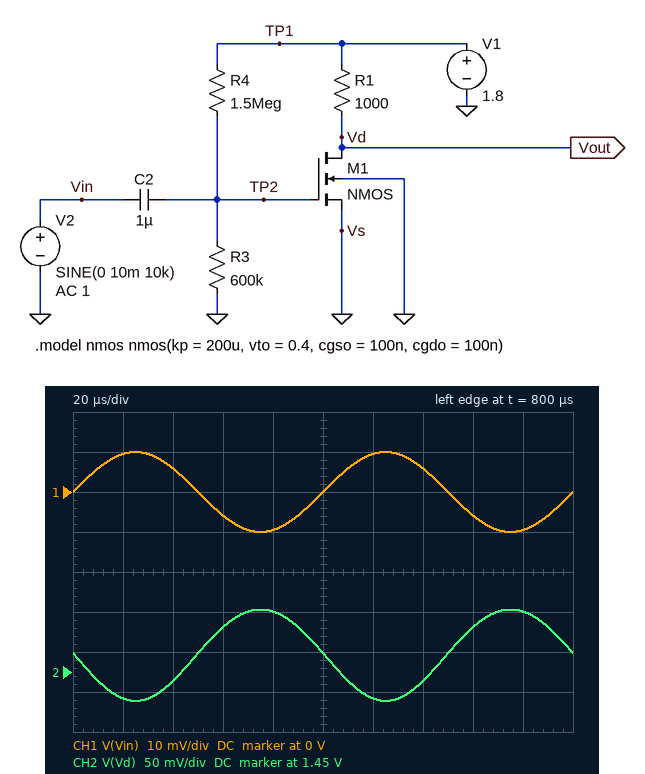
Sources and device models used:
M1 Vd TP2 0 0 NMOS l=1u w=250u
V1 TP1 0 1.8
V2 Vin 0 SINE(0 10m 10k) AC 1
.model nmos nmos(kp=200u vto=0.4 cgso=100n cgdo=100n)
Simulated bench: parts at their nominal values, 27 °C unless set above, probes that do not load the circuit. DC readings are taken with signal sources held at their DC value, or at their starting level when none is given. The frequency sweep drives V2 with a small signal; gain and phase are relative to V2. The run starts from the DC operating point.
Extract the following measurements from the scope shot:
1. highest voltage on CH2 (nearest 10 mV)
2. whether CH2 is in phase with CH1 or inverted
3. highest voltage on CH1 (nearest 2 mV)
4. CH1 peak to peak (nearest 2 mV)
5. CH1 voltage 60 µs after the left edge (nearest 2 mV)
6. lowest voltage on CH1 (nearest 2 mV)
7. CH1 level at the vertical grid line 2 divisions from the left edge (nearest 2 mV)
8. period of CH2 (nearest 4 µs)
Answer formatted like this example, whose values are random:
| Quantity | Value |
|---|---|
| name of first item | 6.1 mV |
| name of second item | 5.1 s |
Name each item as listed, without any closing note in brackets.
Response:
| Quantity | Value |
|---|---|
| highest voltage on CH2 | 1.53 V |
| whether CH2 is in phase with CH1 or inverted | inverted |
| highest voltage on CH1 | 10 mV |
| CH1 peak to peak | 20 mV |
| CH1 voltage 60 µs after the left edge | -6 mV |
| lowest voltage on CH1 | -10 mV |
| CH1 level at the vertical grid line 2 divisions from the left edge | 6 mV |
| period of CH2 | 100 µs |
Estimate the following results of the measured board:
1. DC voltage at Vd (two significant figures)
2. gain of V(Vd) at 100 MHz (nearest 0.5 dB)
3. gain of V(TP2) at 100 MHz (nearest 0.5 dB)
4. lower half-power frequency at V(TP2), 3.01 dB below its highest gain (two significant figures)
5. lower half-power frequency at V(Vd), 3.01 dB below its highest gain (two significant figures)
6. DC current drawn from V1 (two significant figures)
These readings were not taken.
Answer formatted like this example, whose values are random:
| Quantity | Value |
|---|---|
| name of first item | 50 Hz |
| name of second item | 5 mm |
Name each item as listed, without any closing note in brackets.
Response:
| Quantity | Value |
|---|---|
| DC voltage at Vd | 1.5 V |
| gain of V(Vd) at 100 MHz | 0.5 dB |
| gain of V(TP2) at 100 MHz | 0 dB |
| lower half-power frequency at V(TP2), 3.01 dB below its highest gain | 370 mHz |
| lower half-power frequency at V(Vd), 3.01 dB below its highest gain | 370 mHz |
| DC current drawn from V1 | 330 µA |
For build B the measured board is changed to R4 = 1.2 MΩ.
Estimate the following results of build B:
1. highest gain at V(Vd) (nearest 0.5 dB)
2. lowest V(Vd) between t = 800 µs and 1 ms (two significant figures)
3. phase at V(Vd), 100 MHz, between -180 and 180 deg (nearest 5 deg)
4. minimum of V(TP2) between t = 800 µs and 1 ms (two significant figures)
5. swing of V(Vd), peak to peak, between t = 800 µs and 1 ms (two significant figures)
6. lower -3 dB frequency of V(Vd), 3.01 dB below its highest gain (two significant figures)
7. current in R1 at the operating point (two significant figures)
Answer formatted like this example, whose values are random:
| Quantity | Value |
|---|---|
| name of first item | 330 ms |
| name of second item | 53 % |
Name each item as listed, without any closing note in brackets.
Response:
| Quantity | Value |
|---|---|
| highest gain at V(Vd) | 20.0 dB |
| lowest V(Vd) between t = 800 µs and 1 ms | 700 mV |
| phase at V(Vd), 100 MHz, between -180 and 180 deg | 35 deg |
| minimum of V(TP2) between t = 800 µs and 1 ms | 590 mV |
| swing of V(Vd), peak to peak, between t = 800 µs and 1 ms | 200 mV |
| lower -3 dB frequency of V(Vd), 3.01 dB below its highest gain | 400 mHz |
| current in R1 at the operating point | 1.0 mA |
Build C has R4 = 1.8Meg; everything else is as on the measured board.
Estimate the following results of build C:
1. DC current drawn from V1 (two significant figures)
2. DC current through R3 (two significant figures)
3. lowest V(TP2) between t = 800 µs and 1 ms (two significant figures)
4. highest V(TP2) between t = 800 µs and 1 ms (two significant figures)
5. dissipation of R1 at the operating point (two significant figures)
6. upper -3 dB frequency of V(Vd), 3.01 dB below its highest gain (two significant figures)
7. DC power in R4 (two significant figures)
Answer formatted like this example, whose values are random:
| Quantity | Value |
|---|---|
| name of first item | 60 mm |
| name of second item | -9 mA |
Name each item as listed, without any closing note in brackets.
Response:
| Quantity | Value |
|---|---|
| DC current drawn from V1 | 63 µA |
| DC current through R3 | 750 nA |
| lowest V(TP2) between t = 800 µs and 1 ms | 440 mV |
| highest V(TP2) between t = 800 µs and 1 ms | 460 mV |
| dissipation of R1 at the operating point | 3.9 µW |
| upper -3 dB frequency of V(Vd), 3.01 dB below its highest gain | 7.7 MHz |
| DC power in R4 | 1.0 µW |
